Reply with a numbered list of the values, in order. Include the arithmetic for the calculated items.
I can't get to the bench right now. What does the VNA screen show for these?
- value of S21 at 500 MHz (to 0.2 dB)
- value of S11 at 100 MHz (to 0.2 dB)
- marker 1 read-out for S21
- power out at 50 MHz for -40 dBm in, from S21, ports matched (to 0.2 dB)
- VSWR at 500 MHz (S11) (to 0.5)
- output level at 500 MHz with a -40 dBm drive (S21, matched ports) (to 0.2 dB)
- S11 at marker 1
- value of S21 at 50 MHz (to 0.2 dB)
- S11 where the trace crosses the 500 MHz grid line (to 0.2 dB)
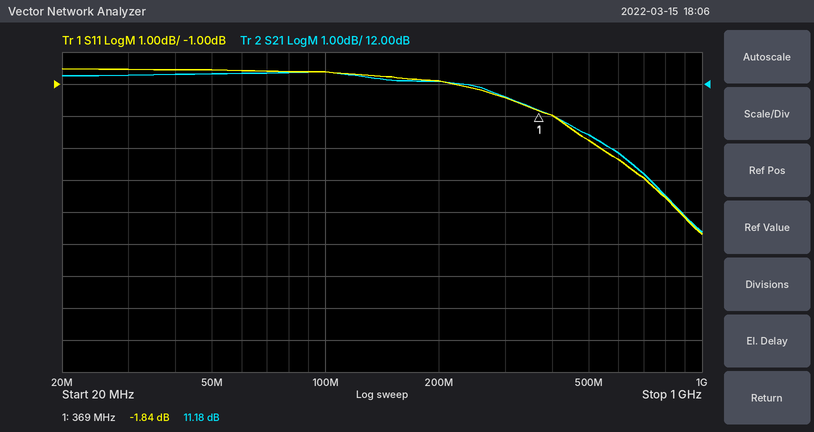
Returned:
1. 10.4 dB
2. -0.6 dB
3. 11.18 dB
4. -40 dBm + (12.4 dB) = -27.6 dBm
5. |Γ| = 10^(-2.8/20) = 0.7244; VSWR = (1 + 0.7244)/(1 − 0.7244) ≈ 6.26, so 6.5 to the nearest 0.5
6. -40 dBm + (10.4 dB) = -29.6 dBm
7. -1.84 dB
8. 12.4 dB
9. -2.8 dB
